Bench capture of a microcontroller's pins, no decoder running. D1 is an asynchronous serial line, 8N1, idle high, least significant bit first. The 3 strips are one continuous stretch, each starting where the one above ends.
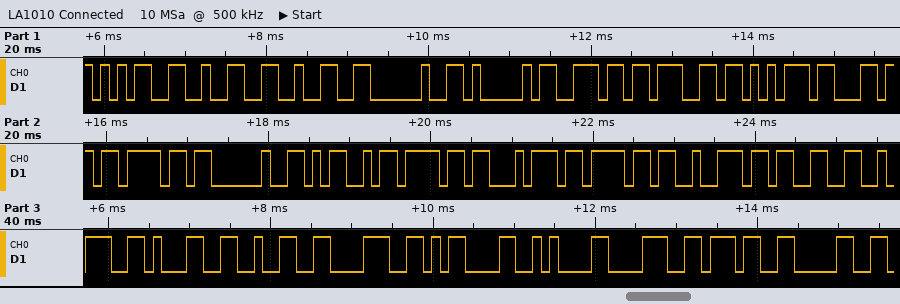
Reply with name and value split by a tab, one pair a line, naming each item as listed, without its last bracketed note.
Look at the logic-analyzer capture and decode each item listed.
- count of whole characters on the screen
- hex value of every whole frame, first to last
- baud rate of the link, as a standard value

count of whole characters on the screen	26
hex value of every whole frame, first to last	35 32 32 20 41 6E 67 75 6C 6F 20 4D 6F 74 6F 72 33 3A 31 32 38 0D 0A 38 37 30
baud rate of the link, as a standard value	9600 baud
